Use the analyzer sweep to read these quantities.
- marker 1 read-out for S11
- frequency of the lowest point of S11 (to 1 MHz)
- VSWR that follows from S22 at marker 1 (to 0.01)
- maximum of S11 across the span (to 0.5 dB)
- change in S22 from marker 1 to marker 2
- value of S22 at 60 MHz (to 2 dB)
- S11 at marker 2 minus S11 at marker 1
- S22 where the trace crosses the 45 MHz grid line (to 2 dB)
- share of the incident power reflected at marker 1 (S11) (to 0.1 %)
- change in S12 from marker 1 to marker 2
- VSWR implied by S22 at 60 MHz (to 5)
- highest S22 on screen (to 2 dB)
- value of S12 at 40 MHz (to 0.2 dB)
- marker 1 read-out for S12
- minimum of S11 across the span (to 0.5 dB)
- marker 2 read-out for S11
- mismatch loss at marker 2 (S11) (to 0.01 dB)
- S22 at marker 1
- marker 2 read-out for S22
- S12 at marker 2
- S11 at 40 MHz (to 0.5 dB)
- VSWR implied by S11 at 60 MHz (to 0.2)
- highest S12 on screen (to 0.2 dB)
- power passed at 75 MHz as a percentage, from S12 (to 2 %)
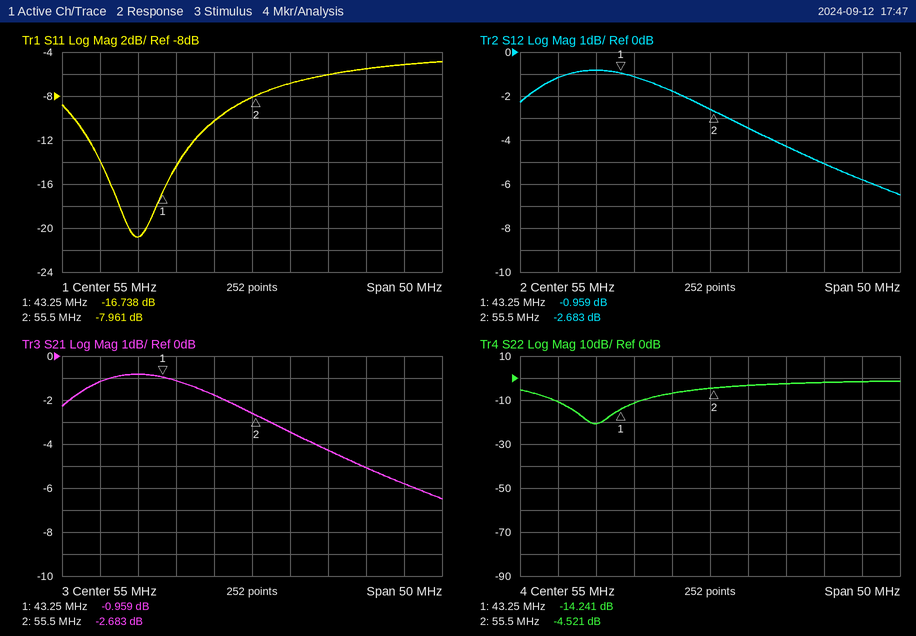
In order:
-16.738 dB
40 MHz
1.48
-5.0 dB
9.720 dB
-4 dB
8.777 dB
-12 dB
2.1 %
-1.724 dB
5
-2 dB
-0.8 dB
-0.959 dB
-21.0 dB
-7.961 dB
0.76 dB
-14.241 dB
-4.521 dB
-2.683 dB
-21.0 dB
2.6
-0.8 dB
26 %
